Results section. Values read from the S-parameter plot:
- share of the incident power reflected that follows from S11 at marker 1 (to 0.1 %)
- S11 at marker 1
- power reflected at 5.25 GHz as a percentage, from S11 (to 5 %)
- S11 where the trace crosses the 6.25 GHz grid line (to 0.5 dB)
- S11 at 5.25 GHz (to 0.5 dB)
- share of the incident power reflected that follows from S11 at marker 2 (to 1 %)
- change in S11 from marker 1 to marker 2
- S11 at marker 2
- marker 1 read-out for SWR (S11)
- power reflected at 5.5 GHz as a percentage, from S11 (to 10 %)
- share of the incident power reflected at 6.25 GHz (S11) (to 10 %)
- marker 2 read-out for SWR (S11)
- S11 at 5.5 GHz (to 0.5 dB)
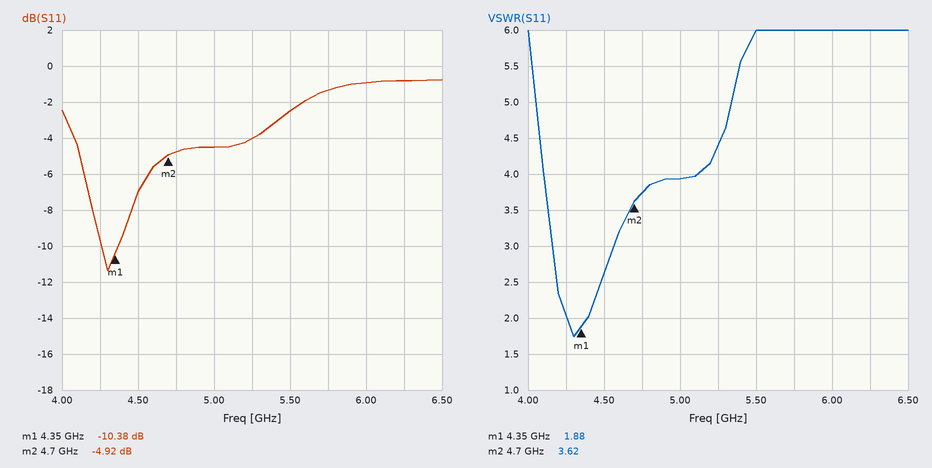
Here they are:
9.2 %
-10.38 dB
40 %
-1.0 dB
-4.0 dB
32 %
5.46 dB
-4.92 dB
1.88
60 %
80 %
3.62
-2.5 dB
